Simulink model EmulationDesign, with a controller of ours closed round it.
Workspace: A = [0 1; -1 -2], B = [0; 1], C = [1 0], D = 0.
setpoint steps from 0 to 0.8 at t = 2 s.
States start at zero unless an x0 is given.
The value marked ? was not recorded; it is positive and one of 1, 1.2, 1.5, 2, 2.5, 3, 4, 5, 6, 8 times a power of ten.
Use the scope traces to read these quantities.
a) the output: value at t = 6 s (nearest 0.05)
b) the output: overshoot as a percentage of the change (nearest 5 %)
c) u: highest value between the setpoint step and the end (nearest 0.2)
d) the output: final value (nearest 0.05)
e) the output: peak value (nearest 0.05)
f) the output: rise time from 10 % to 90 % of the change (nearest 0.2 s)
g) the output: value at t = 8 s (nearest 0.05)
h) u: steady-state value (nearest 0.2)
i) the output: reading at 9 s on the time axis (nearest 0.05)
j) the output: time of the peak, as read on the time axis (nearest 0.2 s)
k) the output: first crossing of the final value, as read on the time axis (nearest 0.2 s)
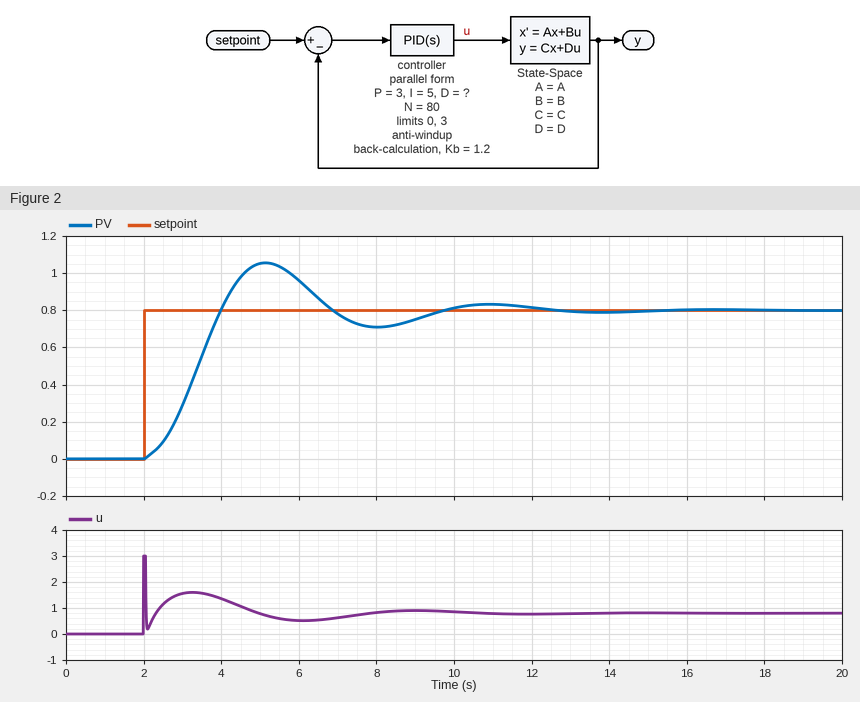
0.95
30 %
3.0
0.80
1.05
1.4 s
0.70
0.8
0.75
5.2 s
4.0 s
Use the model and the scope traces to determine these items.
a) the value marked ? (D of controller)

2.5
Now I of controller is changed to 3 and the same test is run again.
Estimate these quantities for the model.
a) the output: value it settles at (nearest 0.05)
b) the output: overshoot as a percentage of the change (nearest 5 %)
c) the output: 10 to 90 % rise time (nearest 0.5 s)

0.80
15 %
2.0 s
